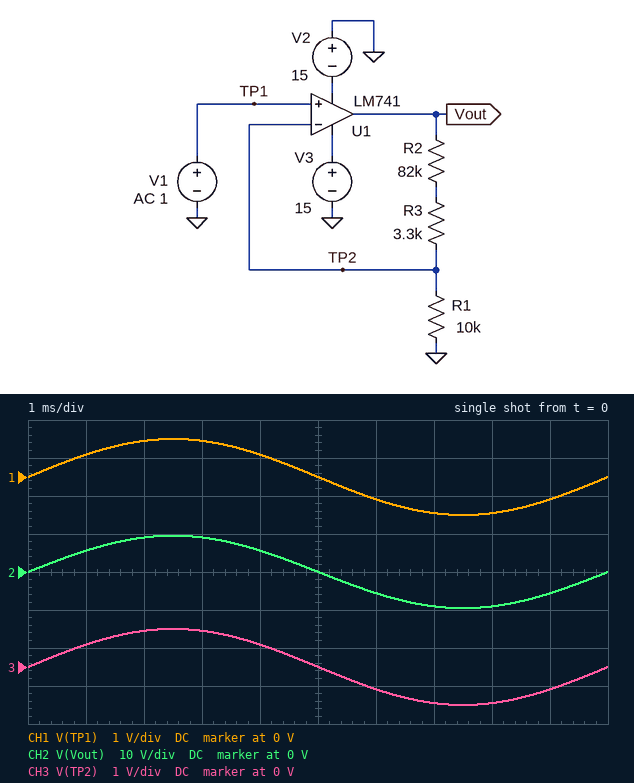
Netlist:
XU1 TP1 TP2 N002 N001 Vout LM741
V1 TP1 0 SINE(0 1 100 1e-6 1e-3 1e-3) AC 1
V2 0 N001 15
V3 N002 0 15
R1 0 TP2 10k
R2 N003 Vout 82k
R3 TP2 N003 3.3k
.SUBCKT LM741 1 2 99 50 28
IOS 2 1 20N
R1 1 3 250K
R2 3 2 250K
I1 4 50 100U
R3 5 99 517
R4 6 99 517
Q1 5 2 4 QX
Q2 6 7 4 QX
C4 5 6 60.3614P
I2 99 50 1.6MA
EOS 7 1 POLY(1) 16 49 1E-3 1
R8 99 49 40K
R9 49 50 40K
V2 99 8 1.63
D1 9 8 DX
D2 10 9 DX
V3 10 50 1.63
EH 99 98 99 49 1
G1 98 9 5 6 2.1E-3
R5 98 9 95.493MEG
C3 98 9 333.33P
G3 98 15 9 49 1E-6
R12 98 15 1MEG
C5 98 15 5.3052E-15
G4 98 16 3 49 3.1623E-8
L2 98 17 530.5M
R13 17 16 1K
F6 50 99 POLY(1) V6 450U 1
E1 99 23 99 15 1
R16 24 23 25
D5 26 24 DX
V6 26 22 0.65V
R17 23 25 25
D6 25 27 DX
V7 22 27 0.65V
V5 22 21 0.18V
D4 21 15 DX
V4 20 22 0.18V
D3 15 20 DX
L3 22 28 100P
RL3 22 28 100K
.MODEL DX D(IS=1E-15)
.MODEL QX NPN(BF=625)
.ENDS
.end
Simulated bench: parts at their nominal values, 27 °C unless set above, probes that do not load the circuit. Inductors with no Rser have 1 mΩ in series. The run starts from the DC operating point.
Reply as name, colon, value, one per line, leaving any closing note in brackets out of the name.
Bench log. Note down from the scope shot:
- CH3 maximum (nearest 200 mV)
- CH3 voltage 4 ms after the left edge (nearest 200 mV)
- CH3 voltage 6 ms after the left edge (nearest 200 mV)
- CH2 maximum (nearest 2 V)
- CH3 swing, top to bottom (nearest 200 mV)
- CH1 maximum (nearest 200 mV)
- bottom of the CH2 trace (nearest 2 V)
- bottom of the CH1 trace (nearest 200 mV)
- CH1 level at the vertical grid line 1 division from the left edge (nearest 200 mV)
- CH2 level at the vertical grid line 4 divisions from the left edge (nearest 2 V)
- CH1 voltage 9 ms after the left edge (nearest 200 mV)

CH3 maximum: 1.0 V
CH3 voltage 4 ms after the left edge: 600 mV
CH3 voltage 6 ms after the left edge: -600 mV
CH2 maximum: 10 V
CH3 swing, top to bottom: 2.0 V
CH1 maximum: 1.0 V
bottom of the CH2 trace: -10 V
bottom of the CH1 trace: -1.0 V
CH1 level at the vertical grid line 1 division from the left edge: 600 mV
CH2 level at the vertical grid line 4 divisions from the left edge: 6 V
CH1 voltage 9 ms after the left edge: -600 mV
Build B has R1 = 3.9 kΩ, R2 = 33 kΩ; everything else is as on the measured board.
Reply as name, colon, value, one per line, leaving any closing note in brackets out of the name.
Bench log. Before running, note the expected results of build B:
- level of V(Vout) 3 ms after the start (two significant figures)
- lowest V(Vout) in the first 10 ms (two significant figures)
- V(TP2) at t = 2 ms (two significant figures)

level of V(Vout) 3 ms after the start: 9.8 V
lowest V(Vout) in the first 10 ms: -10 V
V(TP2) at t = 2 ms: 950 mV
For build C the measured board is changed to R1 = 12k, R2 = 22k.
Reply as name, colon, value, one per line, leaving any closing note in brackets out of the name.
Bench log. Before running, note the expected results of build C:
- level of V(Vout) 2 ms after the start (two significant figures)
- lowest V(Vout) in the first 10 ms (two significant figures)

level of V(Vout) 2 ms after the start: 3.0 V
lowest V(Vout) in the first 10 ms: -3.1 V
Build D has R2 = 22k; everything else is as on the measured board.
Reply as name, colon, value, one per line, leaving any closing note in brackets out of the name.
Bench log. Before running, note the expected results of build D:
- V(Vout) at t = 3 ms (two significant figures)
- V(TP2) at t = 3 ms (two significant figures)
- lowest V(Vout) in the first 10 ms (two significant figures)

V(Vout) at t = 3 ms: 3.4 V
V(TP2) at t = 3 ms: 950 mV
lowest V(Vout) in the first 10 ms: -3.5 V
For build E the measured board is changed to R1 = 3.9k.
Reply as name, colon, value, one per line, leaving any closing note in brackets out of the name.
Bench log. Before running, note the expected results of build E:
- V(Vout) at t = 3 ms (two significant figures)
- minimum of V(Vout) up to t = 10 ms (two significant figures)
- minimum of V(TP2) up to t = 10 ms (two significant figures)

V(Vout) at t = 3 ms: 14 V
minimum of V(Vout) up to t = 10 ms: -14 V
minimum of V(TP2) up to t = 10 ms: -620 mV
